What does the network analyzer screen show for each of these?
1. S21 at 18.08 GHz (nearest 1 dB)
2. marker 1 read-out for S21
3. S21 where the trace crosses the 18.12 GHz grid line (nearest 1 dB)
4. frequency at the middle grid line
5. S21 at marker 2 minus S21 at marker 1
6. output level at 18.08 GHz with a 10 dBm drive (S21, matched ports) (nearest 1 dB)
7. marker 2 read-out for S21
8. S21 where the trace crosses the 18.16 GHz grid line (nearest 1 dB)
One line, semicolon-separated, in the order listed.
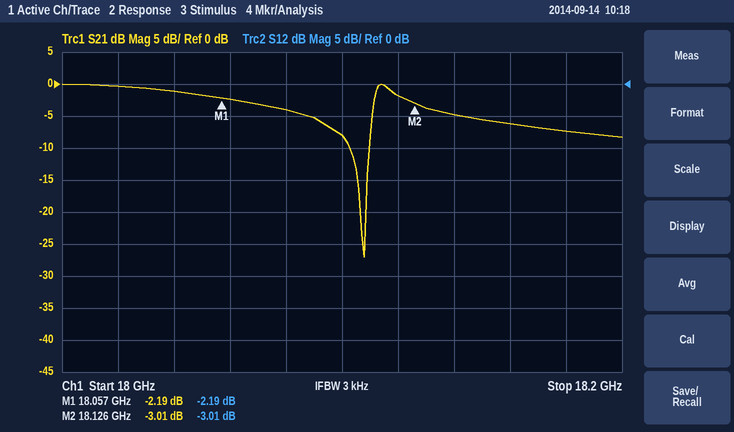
-4 dB; -2.19 dB; -2 dB; 18.1 GHz; -0.82 dB; 6 dBm; -3.01 dB; -6 dB
